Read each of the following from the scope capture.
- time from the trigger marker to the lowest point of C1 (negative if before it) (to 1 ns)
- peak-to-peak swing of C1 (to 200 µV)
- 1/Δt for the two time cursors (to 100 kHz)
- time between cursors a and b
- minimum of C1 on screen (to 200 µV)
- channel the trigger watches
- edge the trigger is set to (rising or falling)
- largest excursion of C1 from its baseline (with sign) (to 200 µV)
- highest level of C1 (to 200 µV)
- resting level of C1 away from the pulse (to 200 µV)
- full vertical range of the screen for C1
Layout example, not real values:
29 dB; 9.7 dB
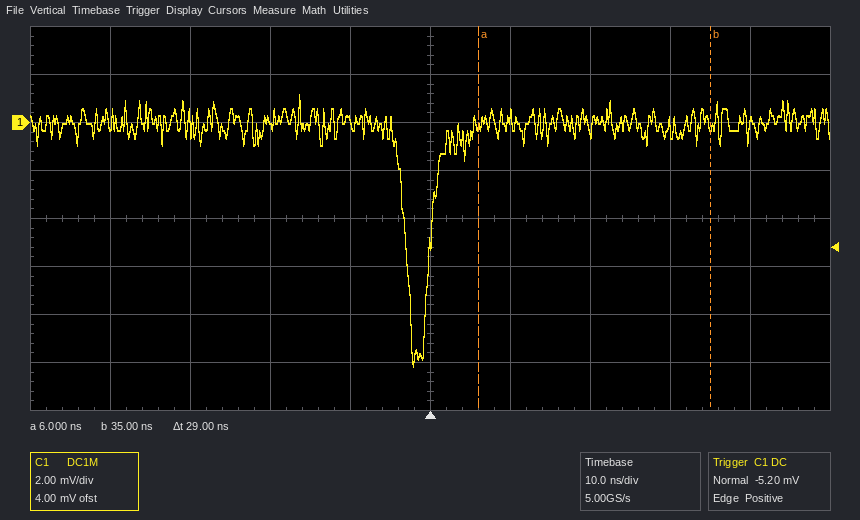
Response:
-2 ns; 11.4 mV; 34.5 MHz; 29 ns; -10.2 mV; C1; rising; -10.2 mV; 1.2 mV; 0.0 mV; 16 mV
